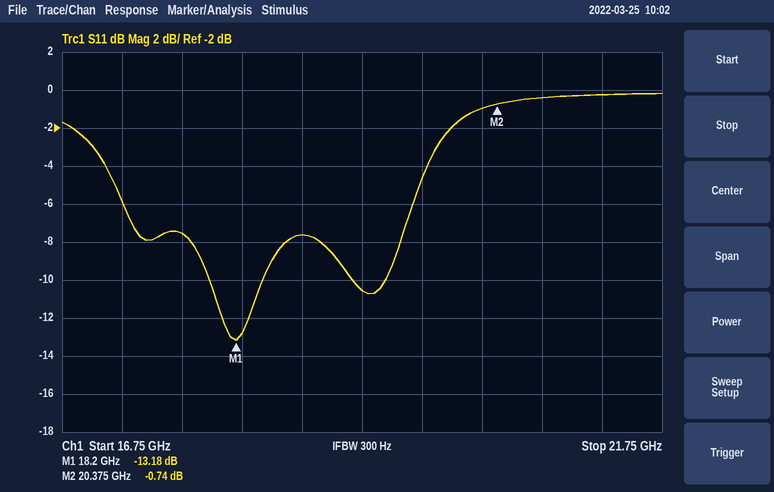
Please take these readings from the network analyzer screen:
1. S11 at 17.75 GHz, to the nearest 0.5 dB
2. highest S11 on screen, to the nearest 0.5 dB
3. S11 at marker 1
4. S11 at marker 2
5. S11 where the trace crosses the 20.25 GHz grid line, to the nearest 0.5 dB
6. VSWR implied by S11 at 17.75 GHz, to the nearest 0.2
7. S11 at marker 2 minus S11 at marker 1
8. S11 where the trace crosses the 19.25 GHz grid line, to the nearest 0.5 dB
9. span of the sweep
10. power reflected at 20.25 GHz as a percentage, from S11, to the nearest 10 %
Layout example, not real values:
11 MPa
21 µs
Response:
-7.5 dB
0.0 dB
-13.18 dB
-0.74 dB
-1.0 dB
2.4
12.44 dB
-10.5 dB
5 GHz
80 %
